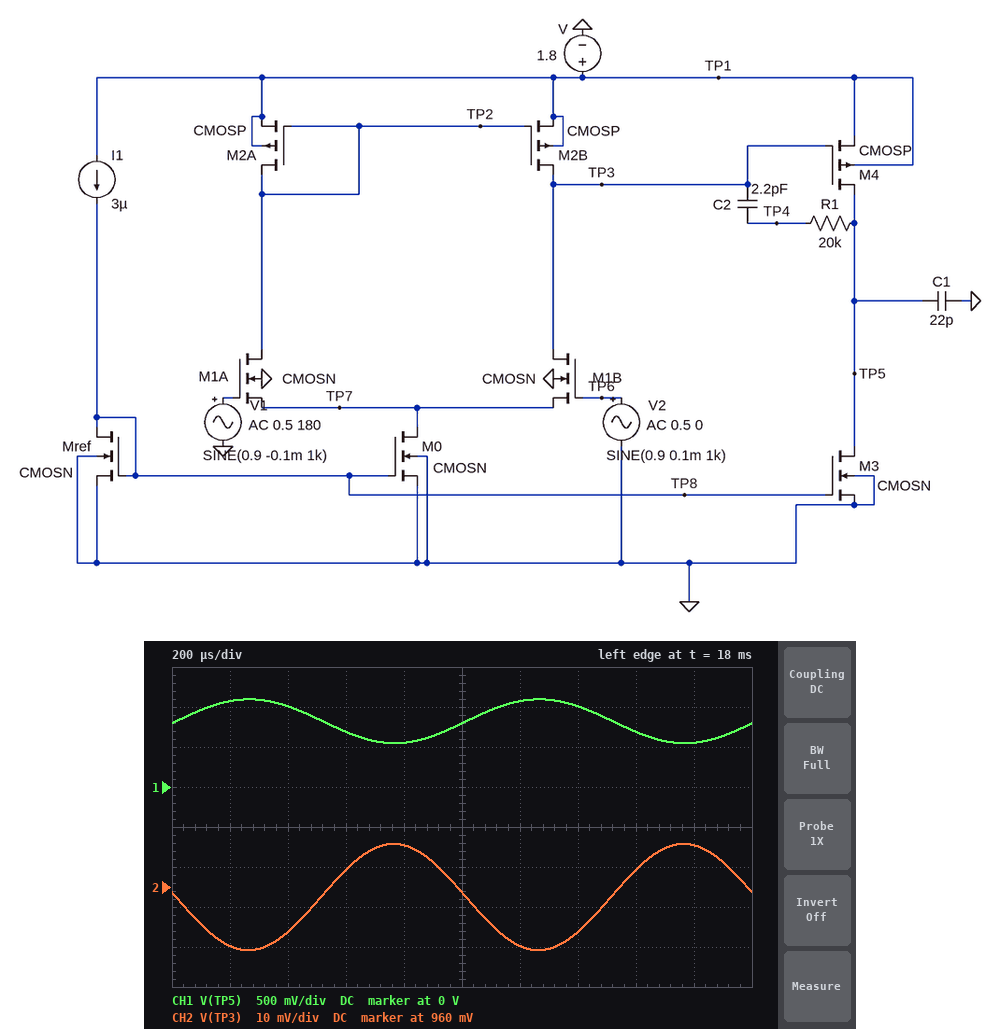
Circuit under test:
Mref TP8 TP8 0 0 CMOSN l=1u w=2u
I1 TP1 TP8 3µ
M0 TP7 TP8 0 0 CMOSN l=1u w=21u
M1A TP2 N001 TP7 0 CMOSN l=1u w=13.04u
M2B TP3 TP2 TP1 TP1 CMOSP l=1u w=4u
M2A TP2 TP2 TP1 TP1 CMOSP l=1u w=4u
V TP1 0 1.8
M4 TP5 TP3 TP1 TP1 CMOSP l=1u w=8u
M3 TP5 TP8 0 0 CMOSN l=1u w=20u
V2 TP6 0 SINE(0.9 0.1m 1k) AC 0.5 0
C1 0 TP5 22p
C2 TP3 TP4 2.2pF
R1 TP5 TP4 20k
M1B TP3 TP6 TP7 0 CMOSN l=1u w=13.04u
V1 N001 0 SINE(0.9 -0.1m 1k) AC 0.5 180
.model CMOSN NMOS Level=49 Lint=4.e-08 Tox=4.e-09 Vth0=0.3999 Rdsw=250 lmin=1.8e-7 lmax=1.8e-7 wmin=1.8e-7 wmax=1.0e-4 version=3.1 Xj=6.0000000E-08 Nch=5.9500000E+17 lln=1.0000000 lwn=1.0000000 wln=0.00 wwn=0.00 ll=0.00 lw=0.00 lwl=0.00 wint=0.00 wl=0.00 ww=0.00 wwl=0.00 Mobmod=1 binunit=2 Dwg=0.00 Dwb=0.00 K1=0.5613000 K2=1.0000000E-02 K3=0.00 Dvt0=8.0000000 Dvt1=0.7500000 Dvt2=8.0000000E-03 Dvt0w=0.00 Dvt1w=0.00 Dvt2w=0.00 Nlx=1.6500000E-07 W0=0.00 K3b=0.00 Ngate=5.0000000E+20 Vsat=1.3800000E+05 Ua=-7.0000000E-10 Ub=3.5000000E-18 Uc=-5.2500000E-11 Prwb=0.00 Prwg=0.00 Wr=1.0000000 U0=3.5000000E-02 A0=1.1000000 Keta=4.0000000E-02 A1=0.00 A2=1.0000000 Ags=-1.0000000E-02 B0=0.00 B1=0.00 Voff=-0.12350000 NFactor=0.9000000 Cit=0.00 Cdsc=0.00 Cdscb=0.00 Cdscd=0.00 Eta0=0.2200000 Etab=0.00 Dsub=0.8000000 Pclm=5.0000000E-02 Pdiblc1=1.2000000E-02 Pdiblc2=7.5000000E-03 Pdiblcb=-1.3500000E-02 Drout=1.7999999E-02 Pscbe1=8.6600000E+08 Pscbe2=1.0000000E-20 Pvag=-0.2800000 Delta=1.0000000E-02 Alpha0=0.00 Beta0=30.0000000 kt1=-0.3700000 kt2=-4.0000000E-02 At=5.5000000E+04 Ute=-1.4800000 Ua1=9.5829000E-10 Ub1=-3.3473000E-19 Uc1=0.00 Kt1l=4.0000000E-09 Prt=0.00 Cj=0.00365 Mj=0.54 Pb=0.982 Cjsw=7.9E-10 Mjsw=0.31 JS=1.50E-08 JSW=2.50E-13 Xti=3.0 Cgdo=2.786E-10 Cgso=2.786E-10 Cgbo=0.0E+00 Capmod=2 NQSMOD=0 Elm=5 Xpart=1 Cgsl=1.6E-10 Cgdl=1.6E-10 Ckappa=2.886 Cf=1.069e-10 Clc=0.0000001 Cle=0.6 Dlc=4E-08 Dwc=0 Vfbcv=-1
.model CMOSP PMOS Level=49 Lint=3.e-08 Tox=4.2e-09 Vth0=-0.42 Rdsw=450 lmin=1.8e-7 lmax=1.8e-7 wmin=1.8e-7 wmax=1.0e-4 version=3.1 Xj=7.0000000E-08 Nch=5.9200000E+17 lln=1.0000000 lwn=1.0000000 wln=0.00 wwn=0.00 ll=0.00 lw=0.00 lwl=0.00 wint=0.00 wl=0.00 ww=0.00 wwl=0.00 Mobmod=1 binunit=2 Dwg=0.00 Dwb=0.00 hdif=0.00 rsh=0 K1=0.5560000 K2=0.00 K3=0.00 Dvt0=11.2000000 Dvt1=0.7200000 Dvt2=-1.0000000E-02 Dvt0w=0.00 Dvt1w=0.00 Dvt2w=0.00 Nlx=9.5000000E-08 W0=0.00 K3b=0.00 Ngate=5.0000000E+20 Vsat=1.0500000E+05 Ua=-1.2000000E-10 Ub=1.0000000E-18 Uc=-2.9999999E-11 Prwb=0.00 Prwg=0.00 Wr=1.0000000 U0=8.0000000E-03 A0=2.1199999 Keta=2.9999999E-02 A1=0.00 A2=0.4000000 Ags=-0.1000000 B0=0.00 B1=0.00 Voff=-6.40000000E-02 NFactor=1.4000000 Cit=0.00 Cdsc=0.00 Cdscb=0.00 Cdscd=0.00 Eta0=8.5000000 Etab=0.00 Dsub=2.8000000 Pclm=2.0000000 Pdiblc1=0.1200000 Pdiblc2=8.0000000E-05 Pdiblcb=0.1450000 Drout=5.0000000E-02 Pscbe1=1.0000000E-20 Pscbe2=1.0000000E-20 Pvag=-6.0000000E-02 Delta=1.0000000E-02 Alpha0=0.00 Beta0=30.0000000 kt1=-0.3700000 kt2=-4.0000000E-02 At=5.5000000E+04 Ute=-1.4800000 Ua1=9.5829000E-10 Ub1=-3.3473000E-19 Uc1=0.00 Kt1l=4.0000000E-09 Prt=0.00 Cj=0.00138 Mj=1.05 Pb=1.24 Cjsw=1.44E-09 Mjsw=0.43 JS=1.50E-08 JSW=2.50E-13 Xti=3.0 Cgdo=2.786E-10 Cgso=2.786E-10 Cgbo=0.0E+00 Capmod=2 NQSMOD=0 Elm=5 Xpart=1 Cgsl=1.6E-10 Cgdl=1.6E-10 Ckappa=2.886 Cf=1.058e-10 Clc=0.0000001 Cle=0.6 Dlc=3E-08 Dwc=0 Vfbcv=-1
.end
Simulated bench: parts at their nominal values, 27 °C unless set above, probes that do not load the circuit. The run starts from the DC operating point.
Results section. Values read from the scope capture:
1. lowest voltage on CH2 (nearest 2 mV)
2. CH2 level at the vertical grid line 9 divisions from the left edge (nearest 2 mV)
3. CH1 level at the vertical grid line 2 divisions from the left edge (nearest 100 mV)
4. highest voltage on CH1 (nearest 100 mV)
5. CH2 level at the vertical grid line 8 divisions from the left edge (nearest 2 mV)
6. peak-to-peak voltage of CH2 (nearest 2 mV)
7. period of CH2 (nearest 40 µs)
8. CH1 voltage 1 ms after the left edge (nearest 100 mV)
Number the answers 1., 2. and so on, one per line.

1. 944 mV
2. 970 mV
3. 1.0 V
4. 1.1 V
5. 964 mV
6. 26 mV
7. 1.00 ms
8. 800 mV
